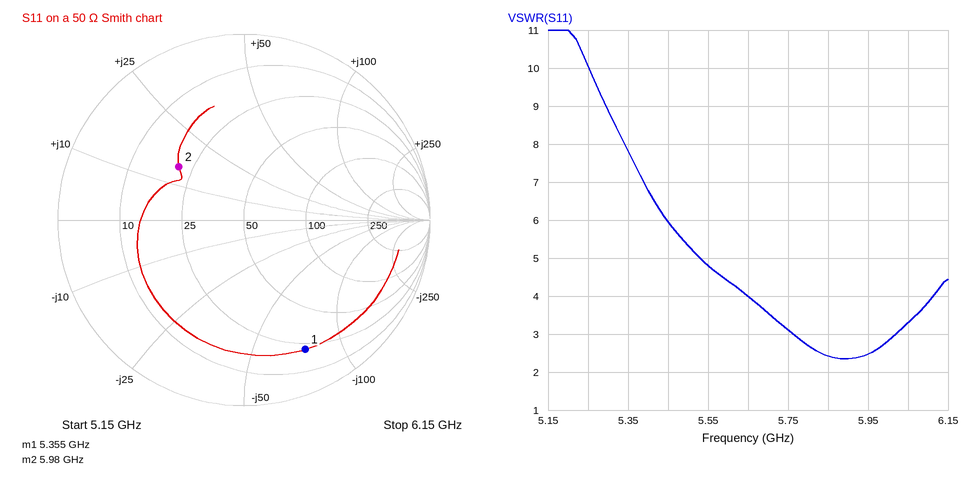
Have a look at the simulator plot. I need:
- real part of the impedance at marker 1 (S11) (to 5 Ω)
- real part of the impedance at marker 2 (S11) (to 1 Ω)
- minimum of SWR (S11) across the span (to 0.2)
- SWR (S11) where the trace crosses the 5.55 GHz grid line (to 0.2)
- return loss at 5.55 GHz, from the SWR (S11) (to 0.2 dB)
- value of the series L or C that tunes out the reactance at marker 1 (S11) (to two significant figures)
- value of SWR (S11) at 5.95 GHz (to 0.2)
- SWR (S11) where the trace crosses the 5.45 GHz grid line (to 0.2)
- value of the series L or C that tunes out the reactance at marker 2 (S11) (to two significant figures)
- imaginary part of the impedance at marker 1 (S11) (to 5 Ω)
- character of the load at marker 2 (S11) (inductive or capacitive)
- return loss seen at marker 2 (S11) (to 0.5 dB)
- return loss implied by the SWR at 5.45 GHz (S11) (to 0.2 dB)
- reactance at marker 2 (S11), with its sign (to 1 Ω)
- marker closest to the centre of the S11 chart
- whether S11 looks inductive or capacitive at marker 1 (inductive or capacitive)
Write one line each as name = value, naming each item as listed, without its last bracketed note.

real part of the impedance at marker 1 (S11) = 20 Ω
real part of the impedance at marker 2 (S11) = 21 Ω
minimum of SWR (S11) across the span = 2.4
SWR (S11) where the trace crosses the 5.55 GHz grid line = 4.8
return loss at 5.55 GHz, from the SWR (S11) = 3.6 dB
value of the series L or C that tunes out the reactance at marker 1 (S11) = 2.2 nH
value of SWR (S11) at 5.95 GHz = 2.4
SWR (S11) where the trace crosses the 5.45 GHz grid line = 6.0
value of the series L or C that tunes out the reactance at marker 2 (S11) = 1.8 pF
imaginary part of the impedance at marker 1 (S11) = -75 Ω
character of the load at marker 2 (S11) = inductive
return loss seen at marker 2 (S11) = 7.0 dB
return loss implied by the SWR at 5.45 GHz (S11) = 3.0 dB
reactance at marker 2 (S11), with its sign = +15 Ω
marker closest to the centre of the S11 chart = marker 2
whether S11 looks inductive or capacitive at marker 1 = capacitive
